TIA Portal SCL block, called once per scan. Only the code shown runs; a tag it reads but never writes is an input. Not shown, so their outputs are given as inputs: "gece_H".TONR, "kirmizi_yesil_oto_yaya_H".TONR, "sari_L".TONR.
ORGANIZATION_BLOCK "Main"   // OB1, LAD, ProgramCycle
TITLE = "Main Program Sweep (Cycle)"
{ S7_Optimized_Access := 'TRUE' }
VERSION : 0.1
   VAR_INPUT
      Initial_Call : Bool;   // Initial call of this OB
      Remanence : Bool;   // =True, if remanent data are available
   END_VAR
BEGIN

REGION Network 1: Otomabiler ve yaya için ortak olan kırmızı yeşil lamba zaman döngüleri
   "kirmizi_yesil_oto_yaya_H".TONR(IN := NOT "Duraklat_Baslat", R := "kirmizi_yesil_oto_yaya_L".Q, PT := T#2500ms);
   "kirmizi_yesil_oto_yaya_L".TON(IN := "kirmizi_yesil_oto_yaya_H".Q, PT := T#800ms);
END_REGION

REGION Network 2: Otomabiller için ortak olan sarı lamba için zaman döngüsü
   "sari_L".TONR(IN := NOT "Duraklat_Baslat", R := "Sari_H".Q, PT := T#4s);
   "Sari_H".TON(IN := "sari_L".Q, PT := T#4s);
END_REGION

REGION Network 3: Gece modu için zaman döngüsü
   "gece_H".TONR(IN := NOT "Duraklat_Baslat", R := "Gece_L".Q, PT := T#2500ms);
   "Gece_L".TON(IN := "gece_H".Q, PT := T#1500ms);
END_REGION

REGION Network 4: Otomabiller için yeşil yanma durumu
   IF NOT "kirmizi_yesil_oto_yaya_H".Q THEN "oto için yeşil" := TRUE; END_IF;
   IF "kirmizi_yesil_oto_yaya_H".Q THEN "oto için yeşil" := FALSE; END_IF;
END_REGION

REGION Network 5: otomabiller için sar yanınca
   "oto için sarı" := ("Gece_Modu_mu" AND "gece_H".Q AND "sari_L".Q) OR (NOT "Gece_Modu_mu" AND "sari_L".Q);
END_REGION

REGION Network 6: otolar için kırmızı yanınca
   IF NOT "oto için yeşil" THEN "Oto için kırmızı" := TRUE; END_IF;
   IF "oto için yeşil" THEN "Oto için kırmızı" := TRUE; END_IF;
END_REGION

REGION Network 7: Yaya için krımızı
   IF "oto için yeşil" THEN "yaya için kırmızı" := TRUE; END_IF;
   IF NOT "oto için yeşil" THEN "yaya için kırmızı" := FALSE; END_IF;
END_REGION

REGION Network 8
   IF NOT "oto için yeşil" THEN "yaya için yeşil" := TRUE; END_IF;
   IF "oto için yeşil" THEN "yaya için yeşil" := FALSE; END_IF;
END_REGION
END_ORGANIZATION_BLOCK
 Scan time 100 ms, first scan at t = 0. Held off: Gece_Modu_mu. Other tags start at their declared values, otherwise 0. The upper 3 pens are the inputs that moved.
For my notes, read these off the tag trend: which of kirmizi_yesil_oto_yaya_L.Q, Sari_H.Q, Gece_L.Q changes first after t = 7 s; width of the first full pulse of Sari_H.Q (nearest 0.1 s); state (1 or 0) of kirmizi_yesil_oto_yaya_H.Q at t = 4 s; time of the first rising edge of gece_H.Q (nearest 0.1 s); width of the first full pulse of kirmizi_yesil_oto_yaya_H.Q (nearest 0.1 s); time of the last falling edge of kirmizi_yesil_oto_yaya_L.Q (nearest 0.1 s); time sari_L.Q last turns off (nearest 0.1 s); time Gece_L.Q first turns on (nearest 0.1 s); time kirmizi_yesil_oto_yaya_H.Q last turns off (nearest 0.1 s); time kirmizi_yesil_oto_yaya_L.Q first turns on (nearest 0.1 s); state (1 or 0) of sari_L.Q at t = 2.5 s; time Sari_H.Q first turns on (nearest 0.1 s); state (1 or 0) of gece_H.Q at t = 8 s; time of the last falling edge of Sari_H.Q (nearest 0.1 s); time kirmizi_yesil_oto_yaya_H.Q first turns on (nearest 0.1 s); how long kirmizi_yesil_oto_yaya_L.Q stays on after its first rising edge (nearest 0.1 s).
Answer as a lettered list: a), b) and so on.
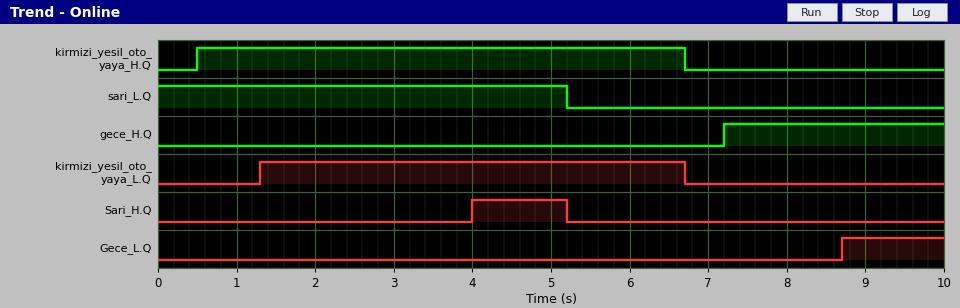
a) Gece_L.Q
b) 1.2 s
c) 1
d) 7.2 s
e) 6.2 s
f) 6.7 s
g) 5.2 s
h) 8.7 s
i) 6.7 s
j) 1.3 s
k) 1
l) 4.0 s
m) 1
n) 5.2 s
o) 0.5 s
p) 5.4 s
